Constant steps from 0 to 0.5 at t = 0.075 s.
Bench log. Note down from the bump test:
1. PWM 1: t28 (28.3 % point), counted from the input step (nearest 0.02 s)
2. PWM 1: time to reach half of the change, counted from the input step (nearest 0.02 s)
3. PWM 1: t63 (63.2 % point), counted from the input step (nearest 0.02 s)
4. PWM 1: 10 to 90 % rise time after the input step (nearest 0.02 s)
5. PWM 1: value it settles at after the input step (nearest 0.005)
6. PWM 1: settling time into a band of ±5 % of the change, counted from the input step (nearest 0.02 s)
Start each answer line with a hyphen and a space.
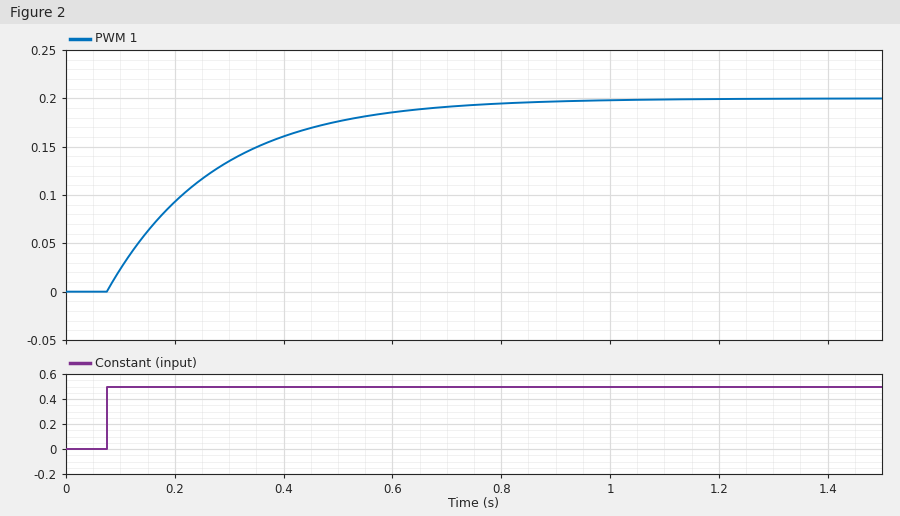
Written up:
- 0.06 s
- 0.14 s
- 0.20 s
- 0.44 s
- 0.200
- 0.60 s
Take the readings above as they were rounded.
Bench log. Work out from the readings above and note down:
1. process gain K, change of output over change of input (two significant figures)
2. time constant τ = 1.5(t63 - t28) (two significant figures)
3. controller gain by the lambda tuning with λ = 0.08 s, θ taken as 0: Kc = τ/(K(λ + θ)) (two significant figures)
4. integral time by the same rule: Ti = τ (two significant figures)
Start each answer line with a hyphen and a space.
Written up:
- 0.40
- 0.21 s
- 6.6
- 0.21 s
